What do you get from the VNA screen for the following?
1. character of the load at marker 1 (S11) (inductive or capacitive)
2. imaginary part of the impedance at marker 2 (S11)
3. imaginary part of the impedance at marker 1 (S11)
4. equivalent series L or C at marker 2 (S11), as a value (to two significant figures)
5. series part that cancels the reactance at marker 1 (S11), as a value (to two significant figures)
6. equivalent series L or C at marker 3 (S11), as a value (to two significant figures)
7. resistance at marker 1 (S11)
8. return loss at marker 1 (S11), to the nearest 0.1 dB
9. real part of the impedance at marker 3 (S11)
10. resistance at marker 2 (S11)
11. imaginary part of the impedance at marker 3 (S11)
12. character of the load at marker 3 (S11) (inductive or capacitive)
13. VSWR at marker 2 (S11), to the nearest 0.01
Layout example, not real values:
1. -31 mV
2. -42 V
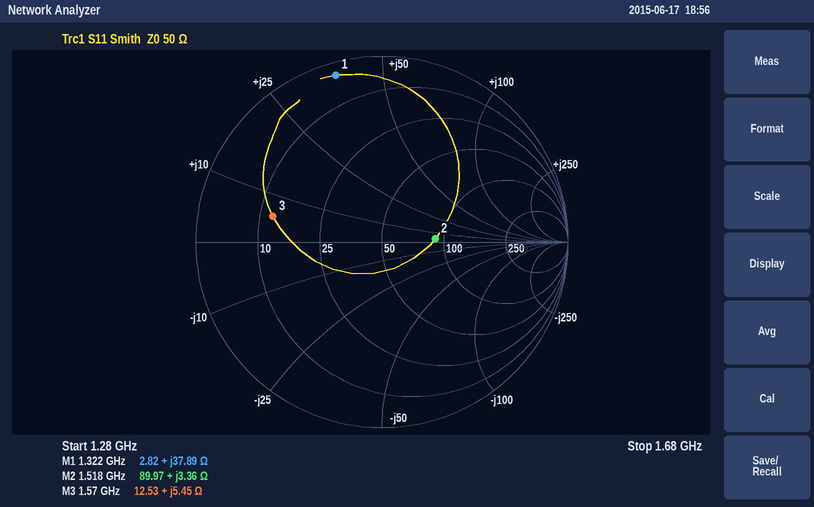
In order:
1. inductive
2. +3.36 Ω
3. +37.89 Ω
4. 350 pH
5. 3.2 pF
6. 550 pH
7. 2.82 Ω
8. 0.6 dB
9. 12.53 Ω
10. 89.97 Ω
11. +5.45 Ω
12. inductive
13. 1.80
